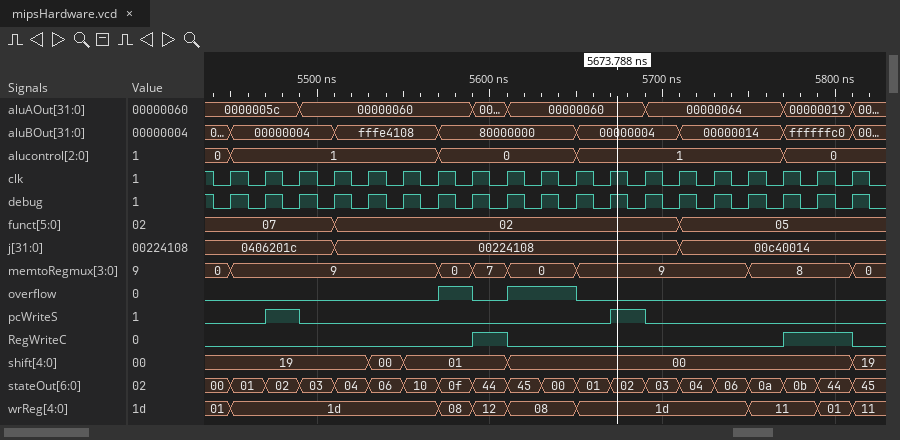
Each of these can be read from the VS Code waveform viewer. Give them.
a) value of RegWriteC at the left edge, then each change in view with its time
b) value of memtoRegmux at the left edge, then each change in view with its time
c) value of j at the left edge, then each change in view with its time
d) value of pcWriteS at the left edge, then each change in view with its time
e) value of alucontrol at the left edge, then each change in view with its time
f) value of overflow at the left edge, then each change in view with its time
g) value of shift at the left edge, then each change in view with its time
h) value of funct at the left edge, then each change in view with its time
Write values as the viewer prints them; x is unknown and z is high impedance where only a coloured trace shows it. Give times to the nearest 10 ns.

0, 1 at 5590 ns, 0 at 5610 ns, 1 at 5770 ns, 0 at 5810 ns
0, 9 at 5450 ns, 0 at 5570 ns, 7 at 5590 ns, 0 at 5610 ns, 9 at 5650 ns, 8 at 5750 ns, 0 at 5810 ns
0406201c, 00224108 at 5510 ns, 00c40014 at 5710 ns
0, 1 at 5470 ns, 0 at 5490 ns, 1 at 5670 ns, 0 at 5690 ns
0, 1 at 5450 ns, 0 at 5570 ns, 1 at 5650 ns, 0 at 5770 ns
0, 1 at 5570 ns, 0 at 5590 ns, 1 at 5610 ns, 0 at 5650 ns
19, 00 at 5530 ns, 01 at 5550 ns, 00 at 5610 ns, 19 at 5810 ns
07, 02 at 5510 ns, 05 at 5710 ns
